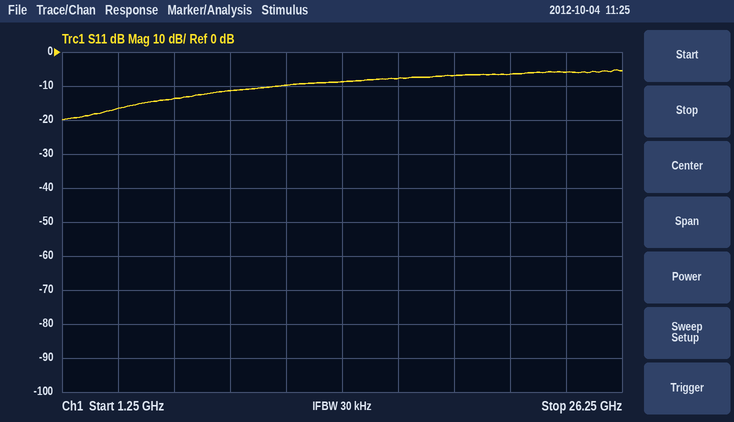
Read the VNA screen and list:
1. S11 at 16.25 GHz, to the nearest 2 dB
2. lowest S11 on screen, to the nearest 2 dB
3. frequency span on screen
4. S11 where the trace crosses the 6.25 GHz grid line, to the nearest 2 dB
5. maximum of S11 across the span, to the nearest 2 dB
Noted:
-8 dB
-20 dB
25 GHz
-14 dB
-6 dB
